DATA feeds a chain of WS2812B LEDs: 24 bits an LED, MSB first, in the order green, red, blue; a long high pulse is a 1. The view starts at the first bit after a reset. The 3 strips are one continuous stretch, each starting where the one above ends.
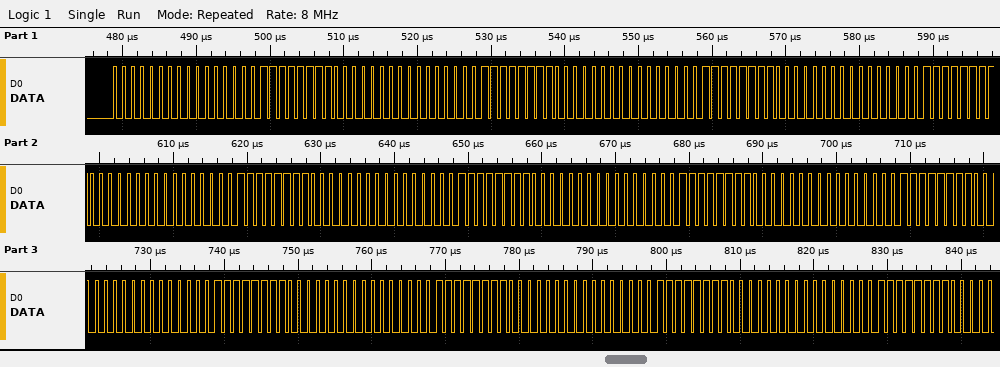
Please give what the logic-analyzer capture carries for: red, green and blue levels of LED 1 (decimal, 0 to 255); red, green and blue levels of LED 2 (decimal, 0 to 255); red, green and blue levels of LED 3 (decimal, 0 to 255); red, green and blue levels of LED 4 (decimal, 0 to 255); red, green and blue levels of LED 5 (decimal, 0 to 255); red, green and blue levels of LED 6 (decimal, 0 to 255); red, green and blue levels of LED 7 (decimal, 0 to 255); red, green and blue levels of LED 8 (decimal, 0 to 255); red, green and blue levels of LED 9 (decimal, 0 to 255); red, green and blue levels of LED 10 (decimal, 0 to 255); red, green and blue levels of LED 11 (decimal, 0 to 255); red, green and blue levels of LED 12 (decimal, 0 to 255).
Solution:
0, 0, 255
0, 0, 255
0, 0, 255
0, 0, 255
0, 0, 255
0, 0, 255
0, 0, 255
0, 0, 255
0, 0, 255
0, 0, 255
0, 0, 255
0, 0, 255
